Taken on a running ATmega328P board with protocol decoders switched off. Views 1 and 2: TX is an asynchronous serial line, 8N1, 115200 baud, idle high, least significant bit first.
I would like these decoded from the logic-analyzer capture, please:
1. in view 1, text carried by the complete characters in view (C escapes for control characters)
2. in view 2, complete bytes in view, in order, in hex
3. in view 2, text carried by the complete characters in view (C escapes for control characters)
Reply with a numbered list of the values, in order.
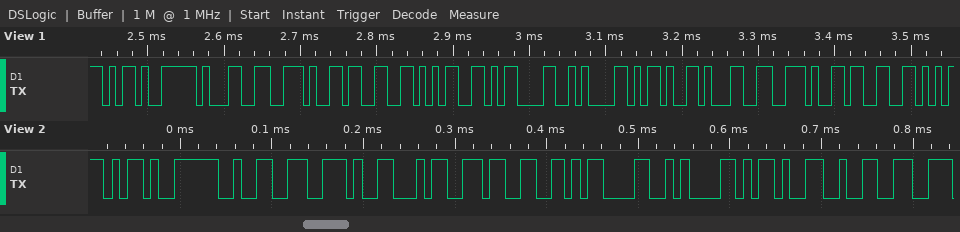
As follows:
1. "-1.35\r\n-1.3"
2. 2D 32 2E 34 33 0D 0A 2D 32
3. "-2.43\r\n-2"
